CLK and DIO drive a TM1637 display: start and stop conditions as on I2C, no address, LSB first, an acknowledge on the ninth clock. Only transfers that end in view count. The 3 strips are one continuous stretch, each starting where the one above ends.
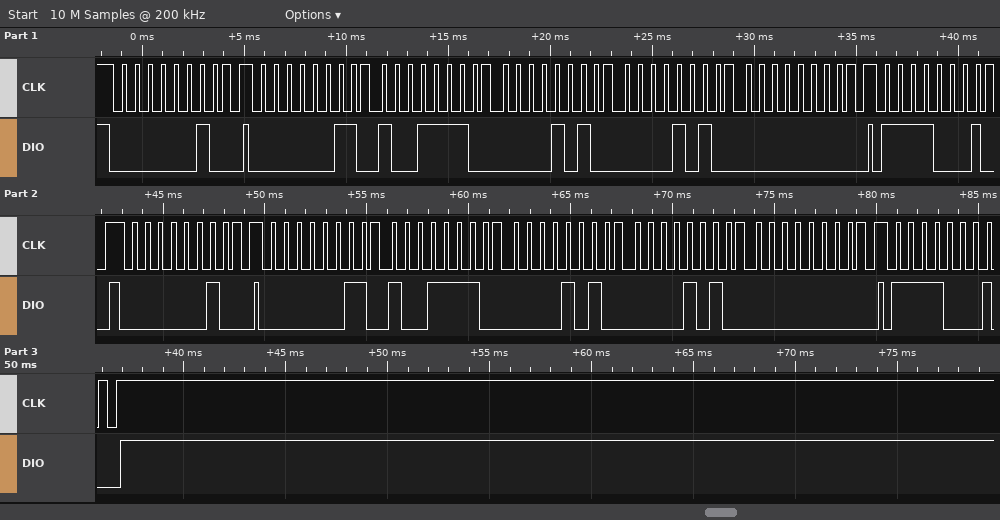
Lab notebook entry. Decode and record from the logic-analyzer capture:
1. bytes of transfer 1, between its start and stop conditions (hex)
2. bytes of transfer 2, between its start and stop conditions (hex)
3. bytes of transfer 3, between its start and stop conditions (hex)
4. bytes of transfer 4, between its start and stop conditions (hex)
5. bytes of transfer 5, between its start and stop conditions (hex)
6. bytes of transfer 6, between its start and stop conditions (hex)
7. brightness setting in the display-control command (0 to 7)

40
C0 79 50 50 00
8F
40
C0 79 50 50 00
8F
7
